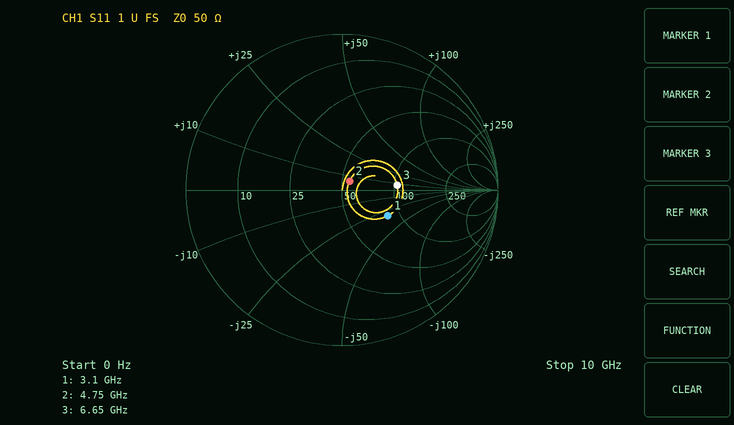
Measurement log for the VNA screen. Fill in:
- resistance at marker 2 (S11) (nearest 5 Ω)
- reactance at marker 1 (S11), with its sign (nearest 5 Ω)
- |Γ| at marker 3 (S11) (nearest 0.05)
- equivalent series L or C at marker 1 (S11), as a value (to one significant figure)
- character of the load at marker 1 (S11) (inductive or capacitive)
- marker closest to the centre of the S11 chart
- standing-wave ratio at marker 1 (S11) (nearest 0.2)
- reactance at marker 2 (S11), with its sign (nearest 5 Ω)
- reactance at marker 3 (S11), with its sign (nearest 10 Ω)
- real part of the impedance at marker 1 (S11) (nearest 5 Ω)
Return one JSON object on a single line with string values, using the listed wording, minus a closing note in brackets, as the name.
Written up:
{"resistance at marker 2 (S11)": "55 Ω", "reactance at marker 1 (S11), with its sign": "-30 Ω", "|Γ| at marker 3 (S11)": "0.35", "equivalent series L or C at marker 1 (S11), as a value": "2 pF", "character of the load at marker 1 (S11)": "capacitive", "marker closest to the centre of the S11 chart": "marker 2", "standing-wave ratio at marker 1 (S11)": "2.0", "reactance at marker 2 (S11), with its sign": "+5 Ω", "reactance at marker 3 (S11), with its sign": "+10 Ω", "real part of the impedance at marker 1 (S11)": "85 Ω"}
